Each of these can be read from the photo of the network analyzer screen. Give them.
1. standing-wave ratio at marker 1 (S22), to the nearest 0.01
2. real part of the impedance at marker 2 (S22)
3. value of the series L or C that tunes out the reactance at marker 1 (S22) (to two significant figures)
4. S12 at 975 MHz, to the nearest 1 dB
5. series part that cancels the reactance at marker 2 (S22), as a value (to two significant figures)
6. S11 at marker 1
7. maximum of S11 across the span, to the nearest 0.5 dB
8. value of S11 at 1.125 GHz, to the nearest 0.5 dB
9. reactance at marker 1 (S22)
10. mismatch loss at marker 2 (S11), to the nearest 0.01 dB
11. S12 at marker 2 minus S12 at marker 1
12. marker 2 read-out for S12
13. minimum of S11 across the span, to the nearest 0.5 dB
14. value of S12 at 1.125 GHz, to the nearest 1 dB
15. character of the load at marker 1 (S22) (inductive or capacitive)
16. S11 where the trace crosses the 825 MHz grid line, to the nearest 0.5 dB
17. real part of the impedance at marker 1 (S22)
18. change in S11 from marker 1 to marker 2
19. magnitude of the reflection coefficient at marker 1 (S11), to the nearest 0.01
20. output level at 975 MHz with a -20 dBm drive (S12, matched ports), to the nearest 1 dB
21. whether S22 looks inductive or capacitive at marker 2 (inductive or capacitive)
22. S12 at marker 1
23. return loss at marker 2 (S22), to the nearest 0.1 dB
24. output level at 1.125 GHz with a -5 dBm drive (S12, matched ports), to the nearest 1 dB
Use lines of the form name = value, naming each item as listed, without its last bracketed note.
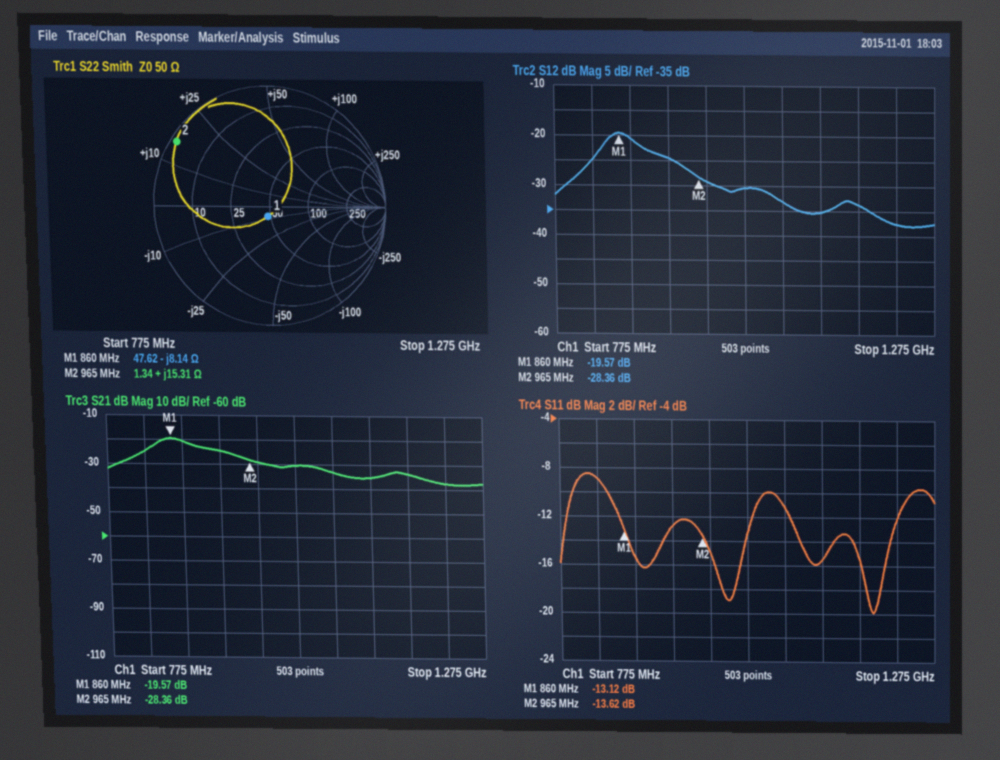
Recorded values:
standing-wave ratio at marker 1 (S22), to the nearest 0.01 = 1.19
real part of the impedance at marker 2 = 1.34 Ω
value of the series L or C that tunes out the reactance at marker 1 (S22) = 1.5 nH
S12 at 975 MHz, to the nearest 1 dB = -29 dB
series part that cancels the reactance at marker 2 (S22), as a value = 11 pF
S11 at marker 1 = -13.12 dB
maximum of S11 across the span, to the nearest 0.5 dB = -8.5 dB
value of S11 at 1.125 GHz, to the nearest 0.5 dB = -15.5 dB
reactance at marker 1 = -8.14 Ω
mismatch loss at marker 2 (S11), to the nearest 0.01 dB = 0.19 dB
S12 at marker 2 minus S12 at marker 1 = -8.79 dB
marker 2 read-out for S12 = -28.36 dB
minimum of S11 across the span, to the nearest 0.5 dB = -20.0 dB
value of S12 at 1.125 GHz, to the nearest 1 dB = -35 dB
character of the load at marker 1 (S22) = capacitive
S11 where the trace crosses the 825 MHz grid line, to the nearest 0.5 dB = -9.0 dB
real part of the impedance at marker 1 = 47.62 Ω
change in S11 from marker 1 to marker 2 = -0.50 dB
magnitude of the reflection coefficient at marker 1 (S11), to the nearest 0.01 = 0.22
output level at 975 MHz with a -20 dBm drive (S12, matched ports), to the nearest 1 dB = -49 dBm
whether S22 looks inductive or capacitive at marker 2 = inductive
S12 at marker 1 = -19.57 dB
return loss at marker 2 (S22), to the nearest 0.1 dB = 0.4 dB
output level at 1.125 GHz with a -5 dBm drive (S12, matched ports), to the nearest 1 dB = -40 dBm
